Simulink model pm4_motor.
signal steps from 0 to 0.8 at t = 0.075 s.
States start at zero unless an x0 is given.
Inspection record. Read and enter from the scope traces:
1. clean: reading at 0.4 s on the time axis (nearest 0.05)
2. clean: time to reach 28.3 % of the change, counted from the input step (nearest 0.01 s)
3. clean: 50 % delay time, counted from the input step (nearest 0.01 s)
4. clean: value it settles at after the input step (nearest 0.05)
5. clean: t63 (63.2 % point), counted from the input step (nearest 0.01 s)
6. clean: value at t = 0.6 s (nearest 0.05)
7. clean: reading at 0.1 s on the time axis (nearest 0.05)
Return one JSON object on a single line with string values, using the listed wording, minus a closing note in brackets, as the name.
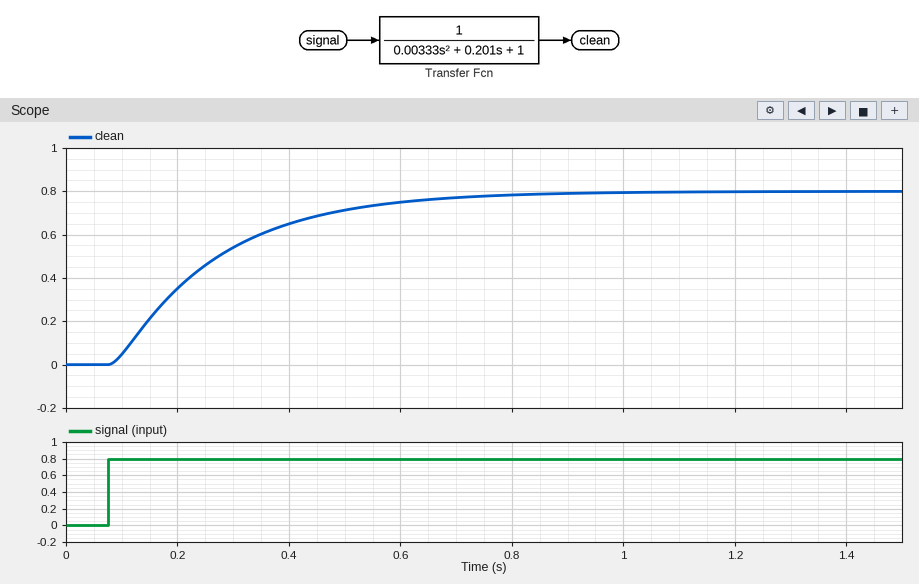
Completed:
{"clean: reading at 0.4 s on the time axis": "0.65", "clean: time to reach 28.3 % of the change, counted from the input step": "0.08 s", "clean: 50 % delay time, counted from the input step": "0.15 s", "clean: value it settles at after the input step": "0.80", "clean: t63 (63.2 % point), counted from the input step": "0.20 s", "clean: value at t = 0.6 s": "0.75", "clean: reading at 0.1 s on the time axis": "0.05"}
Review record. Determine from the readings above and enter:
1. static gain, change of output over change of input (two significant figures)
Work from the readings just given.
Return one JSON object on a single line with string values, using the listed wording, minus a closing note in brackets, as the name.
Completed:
{"static gain, change of output over change of input": "1.0"}
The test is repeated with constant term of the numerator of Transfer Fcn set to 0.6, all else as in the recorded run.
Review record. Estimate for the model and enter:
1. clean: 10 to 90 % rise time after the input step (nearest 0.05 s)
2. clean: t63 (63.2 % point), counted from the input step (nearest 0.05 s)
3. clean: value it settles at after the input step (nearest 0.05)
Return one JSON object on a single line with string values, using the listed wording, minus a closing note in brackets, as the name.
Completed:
{"clean: 10 to 90 % rise time after the input step": "0.40 s", "clean: t63 (63.2 % point), counted from the input step": "0.20 s", "clean: value it settles at after the input step": "0.50"}
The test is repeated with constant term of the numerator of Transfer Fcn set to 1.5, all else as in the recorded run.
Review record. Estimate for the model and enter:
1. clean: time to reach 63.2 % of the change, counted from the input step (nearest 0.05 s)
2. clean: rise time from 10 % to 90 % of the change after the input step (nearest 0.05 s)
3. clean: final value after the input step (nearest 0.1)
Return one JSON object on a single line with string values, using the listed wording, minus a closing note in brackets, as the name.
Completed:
{"clean: time to reach 63.2 % of the change, counted from the input step": "0.20 s", "clean: rise time from 10 % to 90 % of the change after the input step": "0.40 s", "clean: final value after the input step": "1.2"}
